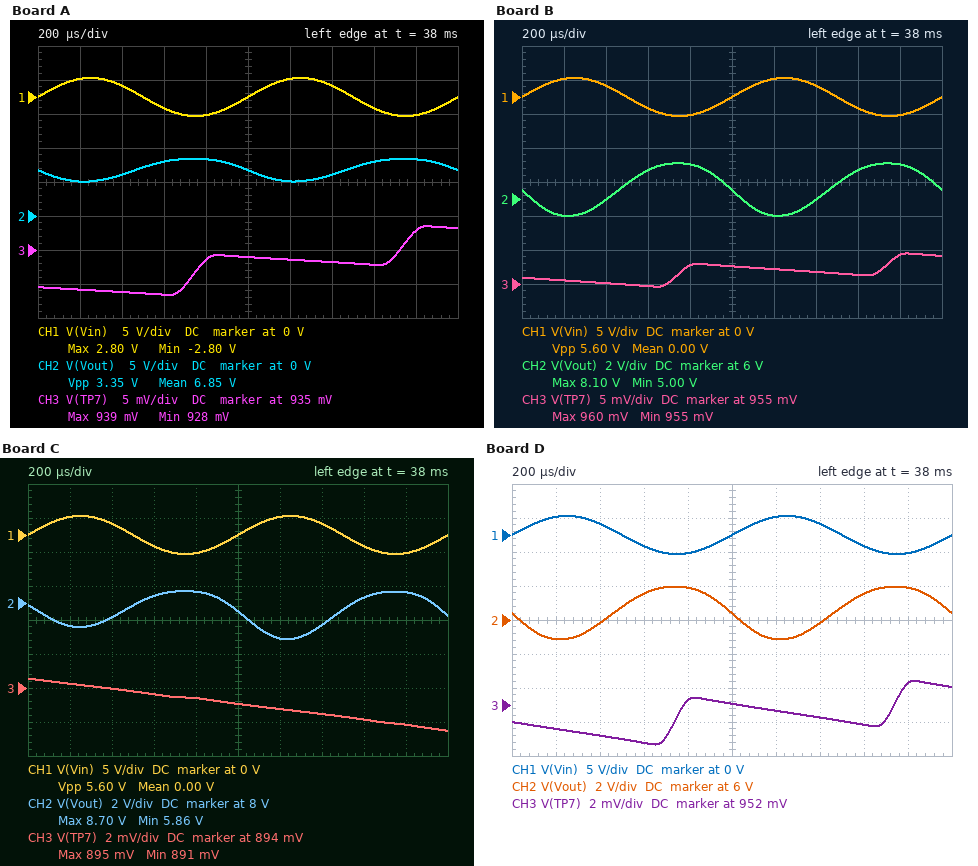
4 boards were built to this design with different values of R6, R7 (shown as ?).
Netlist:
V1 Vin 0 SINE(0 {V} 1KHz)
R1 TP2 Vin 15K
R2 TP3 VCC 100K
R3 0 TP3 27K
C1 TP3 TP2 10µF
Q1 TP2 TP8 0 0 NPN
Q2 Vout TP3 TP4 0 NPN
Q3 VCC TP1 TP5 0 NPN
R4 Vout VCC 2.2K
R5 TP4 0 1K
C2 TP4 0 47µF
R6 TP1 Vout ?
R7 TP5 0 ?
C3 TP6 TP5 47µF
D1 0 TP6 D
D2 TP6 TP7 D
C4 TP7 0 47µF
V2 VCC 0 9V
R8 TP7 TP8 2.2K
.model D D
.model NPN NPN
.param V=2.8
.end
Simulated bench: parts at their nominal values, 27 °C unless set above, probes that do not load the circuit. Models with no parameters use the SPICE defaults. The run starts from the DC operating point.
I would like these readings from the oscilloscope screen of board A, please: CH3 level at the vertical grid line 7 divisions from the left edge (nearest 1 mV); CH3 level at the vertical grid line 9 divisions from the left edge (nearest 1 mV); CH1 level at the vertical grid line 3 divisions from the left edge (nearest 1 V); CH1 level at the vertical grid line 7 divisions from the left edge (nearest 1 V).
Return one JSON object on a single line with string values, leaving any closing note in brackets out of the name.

{"CH3 level at the vertical grid line 7 divisions from the left edge": "933 mV", "CH3 level at the vertical grid line 9 divisions from the left edge": "938 mV", "CH1 level at the vertical grid line 3 divisions from the left edge": "-2 V", "CH1 level at the vertical grid line 7 divisions from the left edge": "2 V"}
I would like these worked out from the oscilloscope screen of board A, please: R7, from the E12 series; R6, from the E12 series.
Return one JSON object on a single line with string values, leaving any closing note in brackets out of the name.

{"R7, from the E12 series": "820 Ω", "R6, from the E12 series": "8.2 kΩ"}
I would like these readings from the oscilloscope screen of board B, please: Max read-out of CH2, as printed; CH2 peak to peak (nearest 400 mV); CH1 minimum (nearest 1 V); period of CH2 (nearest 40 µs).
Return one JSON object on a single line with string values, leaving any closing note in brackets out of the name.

{"Max read-out of CH2, as printed": "8.10 V", "CH2 peak to peak": "3.2 V", "CH1 minimum": "-3 V", "period of CH2": "1.00 ms"}
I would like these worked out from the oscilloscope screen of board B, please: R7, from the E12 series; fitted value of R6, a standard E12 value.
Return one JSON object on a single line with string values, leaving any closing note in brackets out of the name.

{"R7, from the E12 series": "330 Ω", "fitted value of R6, a standard E12 value": "6.8 kΩ"}
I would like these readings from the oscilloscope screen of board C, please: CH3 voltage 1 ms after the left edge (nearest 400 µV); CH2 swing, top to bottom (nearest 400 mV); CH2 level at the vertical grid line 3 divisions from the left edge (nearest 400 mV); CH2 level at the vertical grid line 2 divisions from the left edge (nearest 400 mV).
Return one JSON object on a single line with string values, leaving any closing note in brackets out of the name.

{"CH3 voltage 1 ms after the left edge": "893.2 mV", "CH2 swing, top to bottom": "2.8 V", "CH2 level at the vertical grid line 3 divisions from the left edge": "8.4 V", "CH2 level at the vertical grid line 2 divisions from the left edge": "7.2 V"}
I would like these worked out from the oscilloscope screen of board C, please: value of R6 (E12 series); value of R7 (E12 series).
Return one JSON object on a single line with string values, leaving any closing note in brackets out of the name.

{"value of R6": "27 kΩ", "value of R7": "820 Ω"}
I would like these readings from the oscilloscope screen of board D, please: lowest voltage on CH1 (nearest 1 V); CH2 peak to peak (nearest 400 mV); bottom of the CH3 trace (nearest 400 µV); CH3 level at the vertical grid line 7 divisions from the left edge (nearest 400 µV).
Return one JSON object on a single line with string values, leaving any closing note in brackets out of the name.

{"lowest voltage on CH1": "-3 V", "CH2 peak to peak": "3.2 V", "bottom of the CH3 trace": "949.6 mV", "CH3 level at the vertical grid line 7 divisions from the left edge": "951.2 mV"}
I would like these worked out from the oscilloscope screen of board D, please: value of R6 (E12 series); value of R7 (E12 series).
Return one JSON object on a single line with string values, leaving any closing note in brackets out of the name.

{"value of R6": "5.6 kΩ", "value of R7": "220 Ω"}
